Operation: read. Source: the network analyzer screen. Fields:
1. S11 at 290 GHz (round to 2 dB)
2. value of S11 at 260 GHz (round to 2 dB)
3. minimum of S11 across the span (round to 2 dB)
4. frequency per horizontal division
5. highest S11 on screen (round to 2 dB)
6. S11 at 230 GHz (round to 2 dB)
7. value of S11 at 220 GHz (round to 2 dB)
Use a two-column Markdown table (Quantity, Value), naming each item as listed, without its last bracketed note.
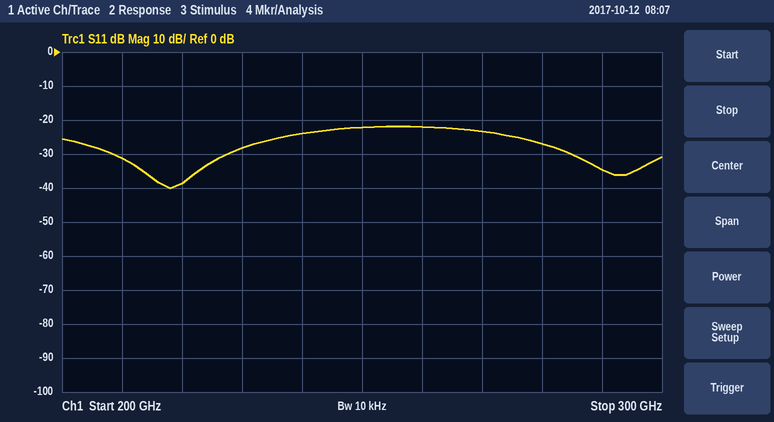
| Quantity | Value |
|---|---|
| S11 at 290 GHz | -34 dB |
| value of S11 at 260 GHz | -22 dB |
| minimum of S11 across the span | -40 dB |
| frequency per horizontal division | 10 GHz |
| highest S11 on screen | -22 dB |
| S11 at 230 GHz | -28 dB |
| value of S11 at 220 GHz | -38 dB |
